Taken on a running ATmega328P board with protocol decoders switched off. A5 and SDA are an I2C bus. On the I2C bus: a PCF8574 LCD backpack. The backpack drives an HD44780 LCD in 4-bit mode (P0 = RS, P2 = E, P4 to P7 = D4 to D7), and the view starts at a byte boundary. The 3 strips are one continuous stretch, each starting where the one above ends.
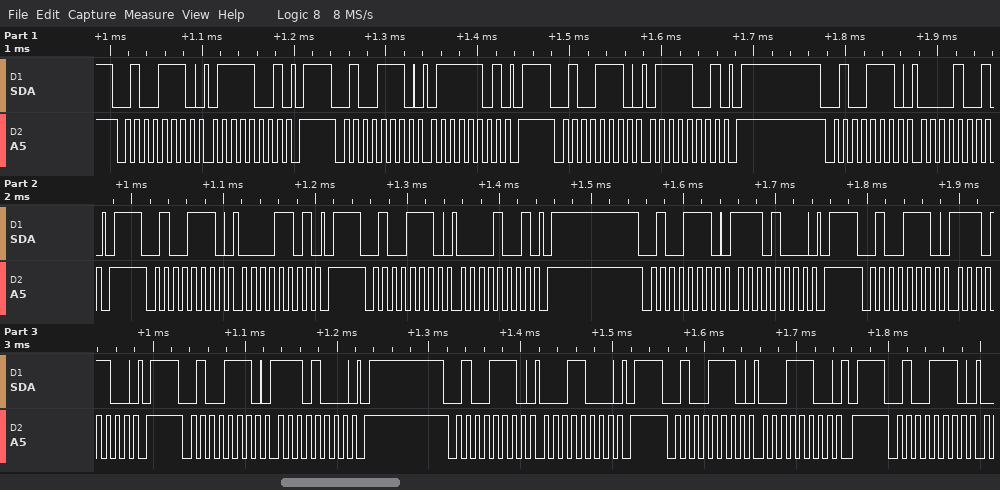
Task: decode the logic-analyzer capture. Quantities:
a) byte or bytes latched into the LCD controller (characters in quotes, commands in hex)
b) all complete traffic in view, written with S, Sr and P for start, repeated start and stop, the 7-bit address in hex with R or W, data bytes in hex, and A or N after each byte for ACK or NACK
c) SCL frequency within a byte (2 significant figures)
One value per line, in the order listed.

'p'
S 27W A 79 A P S 27W A 7D A P S 27W A 79 A P S 27W A 09 A P S 27W A 0D A P S 27W A 09 A P S 27W A E8 A P S 27W A EC A P S 27W A E8 A P S 27W A 18 A P S 27W A 1C A P S 27W A
100 kHz
